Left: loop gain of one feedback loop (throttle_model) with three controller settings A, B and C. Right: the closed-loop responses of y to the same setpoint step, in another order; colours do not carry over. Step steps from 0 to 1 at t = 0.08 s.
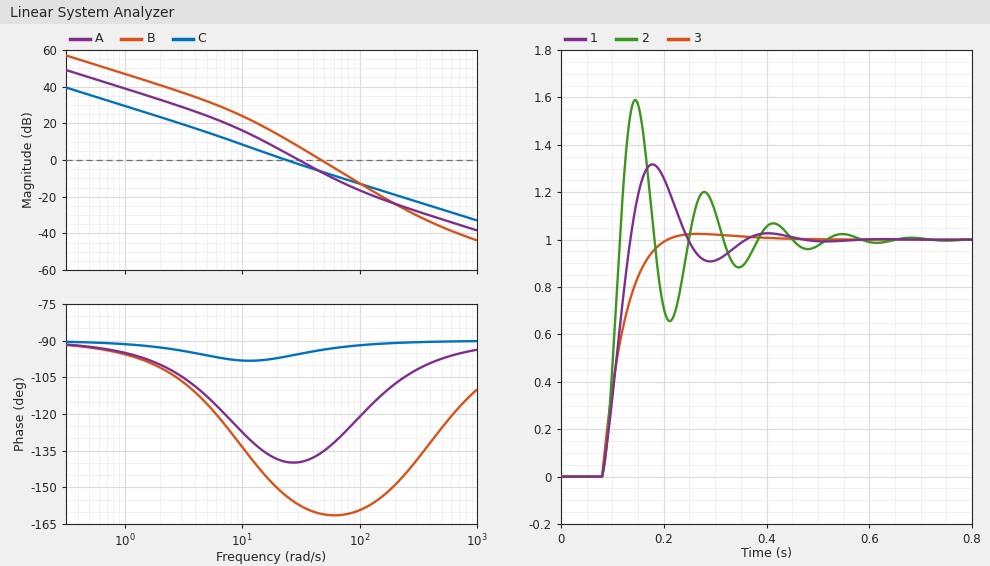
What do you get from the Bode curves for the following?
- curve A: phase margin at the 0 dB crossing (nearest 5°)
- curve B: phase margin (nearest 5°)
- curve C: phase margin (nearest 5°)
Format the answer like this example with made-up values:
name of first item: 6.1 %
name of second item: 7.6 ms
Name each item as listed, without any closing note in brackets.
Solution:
curve A: phase margin at the 0 dB crossing: 40°
curve B: phase margin: 20°
curve C: phase margin: 85°
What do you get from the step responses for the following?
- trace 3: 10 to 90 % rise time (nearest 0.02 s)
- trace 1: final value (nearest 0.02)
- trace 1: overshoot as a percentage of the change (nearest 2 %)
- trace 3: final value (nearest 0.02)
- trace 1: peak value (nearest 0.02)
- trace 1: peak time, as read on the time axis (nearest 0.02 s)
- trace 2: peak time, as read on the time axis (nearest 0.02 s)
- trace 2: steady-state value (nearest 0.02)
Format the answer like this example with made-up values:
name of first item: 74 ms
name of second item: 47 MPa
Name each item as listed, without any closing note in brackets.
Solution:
trace 3: 10 to 90 % rise time: 0.08 s
trace 1: final value: 1.00
trace 1: overshoot as a percentage of the change: 32 %
trace 3: final value: 1.00
trace 1: peak value: 1.32
trace 1: peak time, as read on the time axis: 0.18 s
trace 2: peak time, as read on the time axis: 0.14 s
trace 2: steady-state value: 1.00
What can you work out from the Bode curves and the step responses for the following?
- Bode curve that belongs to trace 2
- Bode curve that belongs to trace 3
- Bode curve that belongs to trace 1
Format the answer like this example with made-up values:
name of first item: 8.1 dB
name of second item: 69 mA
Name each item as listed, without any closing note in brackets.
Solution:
Bode curve that belongs to trace 2: B
Bode curve that belongs to trace 3: C
Bode curve that belongs to trace 1: A
